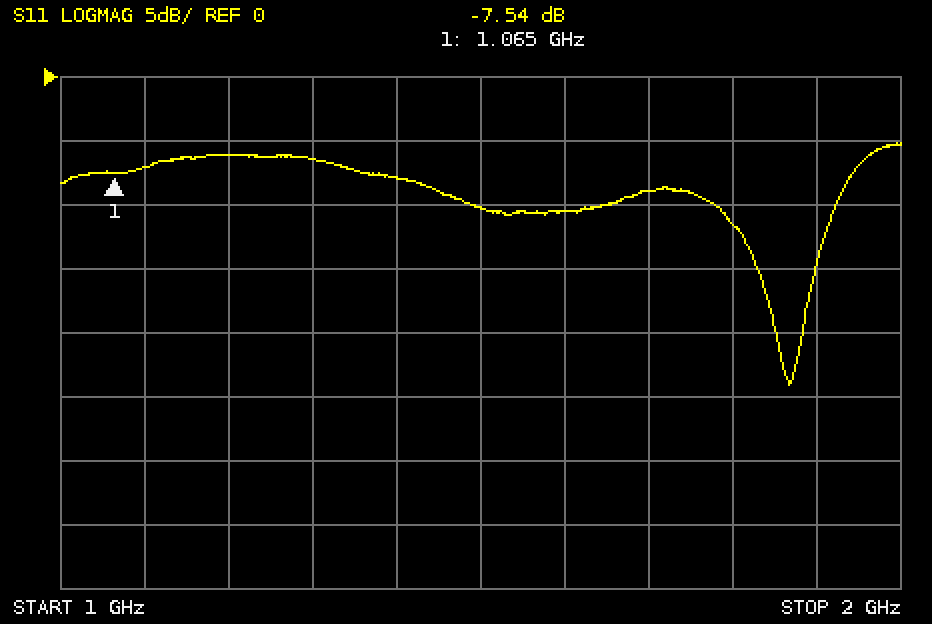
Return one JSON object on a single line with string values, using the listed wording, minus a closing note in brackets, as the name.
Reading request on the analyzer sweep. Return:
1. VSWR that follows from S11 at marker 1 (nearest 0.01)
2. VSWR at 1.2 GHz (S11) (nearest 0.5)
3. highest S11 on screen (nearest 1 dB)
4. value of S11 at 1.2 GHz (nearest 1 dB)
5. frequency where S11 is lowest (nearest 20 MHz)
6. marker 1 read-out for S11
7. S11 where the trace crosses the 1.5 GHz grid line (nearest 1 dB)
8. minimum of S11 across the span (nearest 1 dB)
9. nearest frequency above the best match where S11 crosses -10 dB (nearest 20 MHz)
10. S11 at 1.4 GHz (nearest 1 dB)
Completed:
{"VSWR that follows from S11 at marker 1": "2.45", "VSWR at 1.2 GHz (S11)": "3.0", "highest S11 on screen": "-5 dB", "value of S11 at 1.2 GHz": "-6 dB", "frequency where S11 is lowest": "1.86 GHz", "marker 1 read-out for S11": "-7.54 dB", "S11 where the trace crosses the 1.5 GHz grid line": "-10 dB", "minimum of S11 across the span": "-24 dB", "nearest frequency above the best match where S11 crosses -10 dB": "1.92 GHz", "S11 at 1.4 GHz": "-8 dB"}
